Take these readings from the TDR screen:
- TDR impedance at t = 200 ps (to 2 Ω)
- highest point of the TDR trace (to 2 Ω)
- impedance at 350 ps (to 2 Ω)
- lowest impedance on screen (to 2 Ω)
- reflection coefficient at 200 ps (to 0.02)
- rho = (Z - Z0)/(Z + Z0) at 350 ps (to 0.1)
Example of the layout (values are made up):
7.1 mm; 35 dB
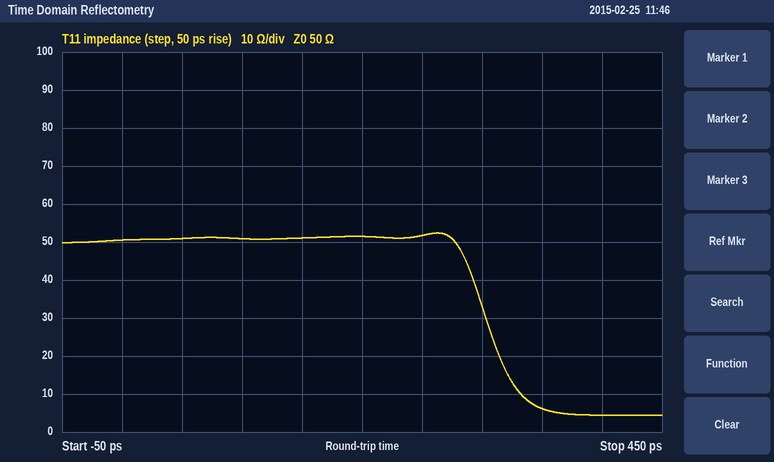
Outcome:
52 Ω; 52 Ω; 6 Ω; 4 Ω; +0.02; -0.8
